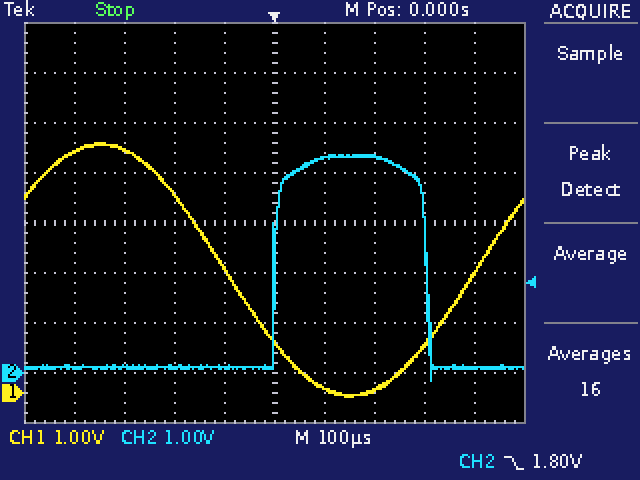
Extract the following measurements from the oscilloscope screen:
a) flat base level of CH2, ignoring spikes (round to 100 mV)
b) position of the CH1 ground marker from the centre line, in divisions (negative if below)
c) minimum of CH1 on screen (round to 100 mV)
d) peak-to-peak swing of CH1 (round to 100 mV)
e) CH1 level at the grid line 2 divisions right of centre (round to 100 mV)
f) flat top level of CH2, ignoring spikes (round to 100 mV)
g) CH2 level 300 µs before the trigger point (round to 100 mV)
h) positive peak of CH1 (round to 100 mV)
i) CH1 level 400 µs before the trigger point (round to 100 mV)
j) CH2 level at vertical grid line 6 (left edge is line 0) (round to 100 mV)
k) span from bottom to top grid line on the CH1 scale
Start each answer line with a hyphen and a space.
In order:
- 100 mV
- -3.4 div
- -100 mV
- 5.1 V
- 100 mV
- 4.3 V
- 100 mV
- 5.0 V
- 4.8 V
- 4.3 V
- 8 V
